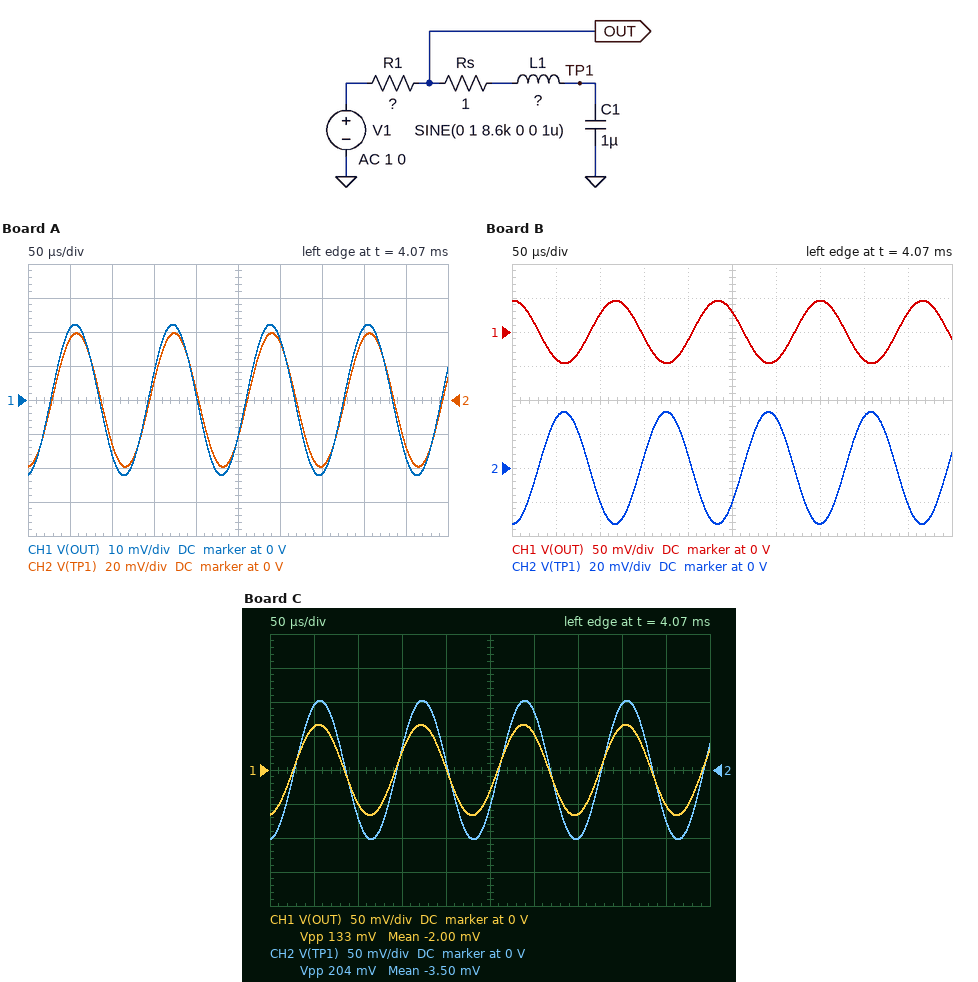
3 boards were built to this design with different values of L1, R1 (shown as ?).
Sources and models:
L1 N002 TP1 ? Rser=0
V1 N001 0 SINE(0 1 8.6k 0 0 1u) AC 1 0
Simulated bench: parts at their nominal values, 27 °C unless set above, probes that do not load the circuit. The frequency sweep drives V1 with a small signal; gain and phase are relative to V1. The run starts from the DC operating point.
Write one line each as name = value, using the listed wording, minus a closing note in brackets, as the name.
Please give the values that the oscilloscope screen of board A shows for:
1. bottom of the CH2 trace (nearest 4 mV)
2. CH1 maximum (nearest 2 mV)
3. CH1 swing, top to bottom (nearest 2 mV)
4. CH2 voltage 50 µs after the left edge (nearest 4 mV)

bottom of the CH2 trace = -40 mV
CH1 maximum = 22 mV
CH1 swing, top to bottom = 44 mV
CH2 voltage 50 µs after the left edge = 36 mV
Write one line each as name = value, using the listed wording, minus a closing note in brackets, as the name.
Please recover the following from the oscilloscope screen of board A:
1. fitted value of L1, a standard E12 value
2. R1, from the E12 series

fitted value of L1, a standard E12 value = 150 µH
R1, from the E12 series = 470 Ω
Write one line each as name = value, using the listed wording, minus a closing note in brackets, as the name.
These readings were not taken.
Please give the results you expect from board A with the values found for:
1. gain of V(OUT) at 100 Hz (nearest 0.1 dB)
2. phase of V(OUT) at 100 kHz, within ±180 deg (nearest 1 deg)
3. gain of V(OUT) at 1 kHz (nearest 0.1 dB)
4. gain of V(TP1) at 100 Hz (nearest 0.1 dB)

gain of V(OUT) at 100 Hz = -0.4 dB
phase of V(OUT) at 100 kHz, within ±180 deg = 78 deg
gain of V(OUT) at 1 kHz = -9.9 dB
gain of V(TP1) at 100 Hz = -0.4 dB
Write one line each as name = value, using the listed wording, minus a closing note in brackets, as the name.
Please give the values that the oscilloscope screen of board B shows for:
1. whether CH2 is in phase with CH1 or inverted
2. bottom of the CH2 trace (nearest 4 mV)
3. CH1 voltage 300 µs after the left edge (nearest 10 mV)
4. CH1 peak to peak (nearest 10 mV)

whether CH2 is in phase with CH1 or inverted = inverted
bottom of the CH2 trace = -32 mV
CH1 voltage 300 µs after the left edge = -40 mV
CH1 peak to peak = 90 mV
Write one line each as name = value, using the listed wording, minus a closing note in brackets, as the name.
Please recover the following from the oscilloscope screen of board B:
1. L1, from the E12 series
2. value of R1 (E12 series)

L1, from the E12 series = 820 µH
value of R1 = 560 Ω
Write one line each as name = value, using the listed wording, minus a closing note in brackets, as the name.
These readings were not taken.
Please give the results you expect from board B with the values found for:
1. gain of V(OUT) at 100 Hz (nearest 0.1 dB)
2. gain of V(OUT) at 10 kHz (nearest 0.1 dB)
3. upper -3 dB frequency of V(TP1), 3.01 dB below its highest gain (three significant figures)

gain of V(OUT) at 100 Hz = -0.5 dB
gain of V(OUT) at 10 kHz = -24.0 dB
upper -3 dB frequency of V(TP1), 3.01 dB below its highest gain = 284 Hz
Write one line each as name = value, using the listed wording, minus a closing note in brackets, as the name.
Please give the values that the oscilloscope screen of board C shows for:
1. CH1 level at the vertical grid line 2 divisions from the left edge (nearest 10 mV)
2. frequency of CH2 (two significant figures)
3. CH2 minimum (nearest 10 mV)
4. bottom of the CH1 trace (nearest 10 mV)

CH1 level at the vertical grid line 2 divisions from the left edge = -50 mV
frequency of CH2 = 8.6 kHz
CH2 minimum = -100 mV
bottom of the CH1 trace = -70 mV
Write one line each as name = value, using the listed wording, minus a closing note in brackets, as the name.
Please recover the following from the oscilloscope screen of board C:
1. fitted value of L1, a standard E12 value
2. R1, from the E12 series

fitted value of L1, a standard E12 value = 120 µH
R1, from the E12 series = 180 Ω
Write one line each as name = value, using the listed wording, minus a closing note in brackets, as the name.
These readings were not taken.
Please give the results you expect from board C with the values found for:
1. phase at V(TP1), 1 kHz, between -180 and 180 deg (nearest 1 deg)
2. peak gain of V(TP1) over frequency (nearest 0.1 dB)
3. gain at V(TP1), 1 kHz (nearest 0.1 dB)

phase at V(TP1), 1 kHz, between -180 and 180 deg = -49 deg
peak gain of V(TP1) over frequency = 0 dB
gain at V(TP1), 1 kHz = -3.6 dB
